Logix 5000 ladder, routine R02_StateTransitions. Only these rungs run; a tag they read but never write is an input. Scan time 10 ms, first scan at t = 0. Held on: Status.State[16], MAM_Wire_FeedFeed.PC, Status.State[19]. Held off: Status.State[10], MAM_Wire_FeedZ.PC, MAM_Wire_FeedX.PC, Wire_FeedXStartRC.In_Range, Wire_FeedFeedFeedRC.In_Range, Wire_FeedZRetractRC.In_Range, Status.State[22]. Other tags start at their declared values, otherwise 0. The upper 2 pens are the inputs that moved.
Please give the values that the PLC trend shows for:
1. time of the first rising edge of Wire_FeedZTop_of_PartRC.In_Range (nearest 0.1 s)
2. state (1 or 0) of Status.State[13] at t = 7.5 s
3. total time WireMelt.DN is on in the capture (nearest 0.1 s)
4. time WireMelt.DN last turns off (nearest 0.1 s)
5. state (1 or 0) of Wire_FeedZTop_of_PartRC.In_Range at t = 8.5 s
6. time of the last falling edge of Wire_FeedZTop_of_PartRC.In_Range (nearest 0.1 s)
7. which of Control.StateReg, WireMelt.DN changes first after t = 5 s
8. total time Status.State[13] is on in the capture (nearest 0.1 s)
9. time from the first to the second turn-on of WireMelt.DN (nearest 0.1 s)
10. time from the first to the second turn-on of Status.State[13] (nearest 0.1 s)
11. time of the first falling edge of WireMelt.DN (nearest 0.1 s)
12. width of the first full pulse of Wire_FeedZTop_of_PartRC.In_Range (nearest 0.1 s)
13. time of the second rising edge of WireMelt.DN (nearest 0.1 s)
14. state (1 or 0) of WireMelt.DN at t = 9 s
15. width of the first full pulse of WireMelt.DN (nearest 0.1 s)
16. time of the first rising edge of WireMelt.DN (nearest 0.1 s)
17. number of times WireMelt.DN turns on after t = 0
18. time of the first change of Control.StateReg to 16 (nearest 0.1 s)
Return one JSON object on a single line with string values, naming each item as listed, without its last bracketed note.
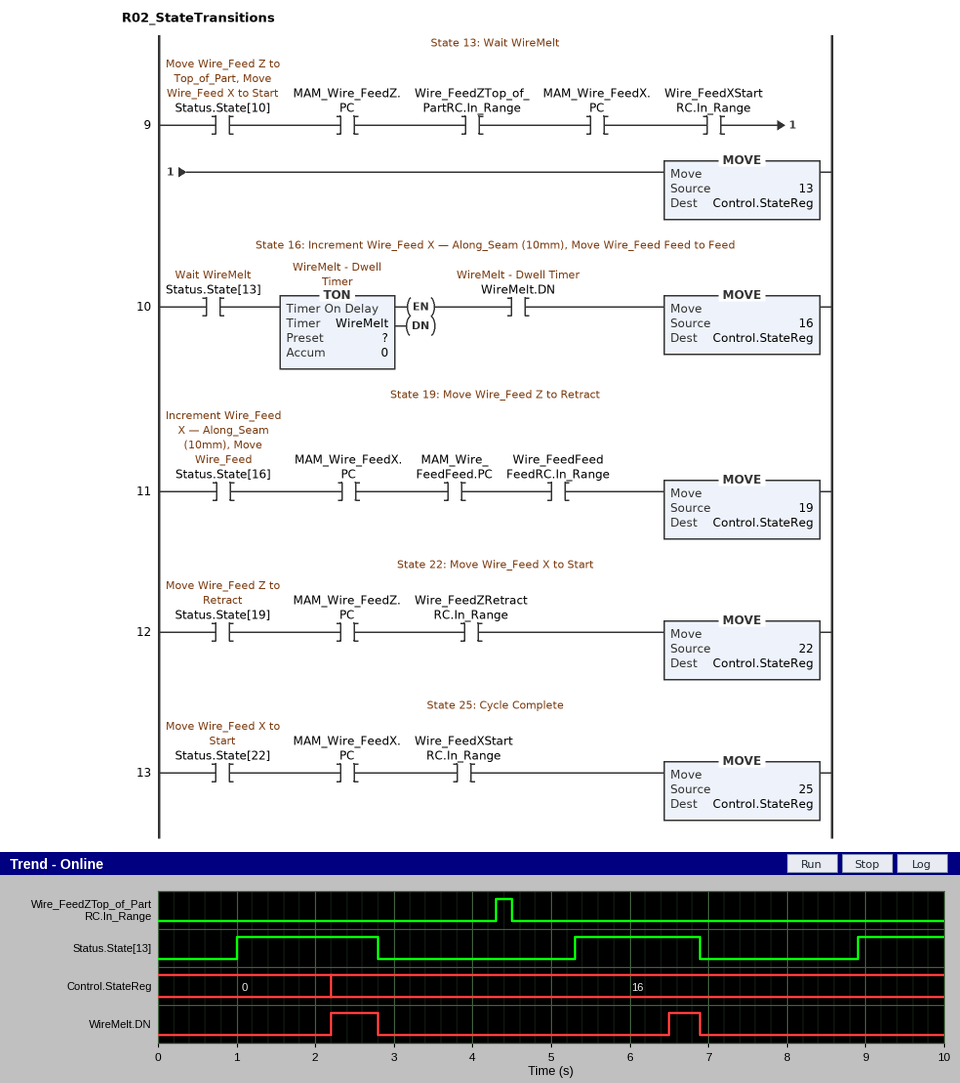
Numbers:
{"time of the first rising edge of Wire_FeedZTop_of_PartRC.In_Range": "4.3 s", "state (1 or 0) of Status.State[13] at t = 7.5 s": "0", "total time WireMelt.DN is on in the capture": "1.0 s", "time WireMelt.DN last turns off": "6.9 s", "state (1 or 0) of Wire_FeedZTop_of_PartRC.In_Range at t = 8.5 s": "0", "time of the last falling edge of Wire_FeedZTop_of_PartRC.In_Range": "4.5 s", "which of Control.StateReg, WireMelt.DN changes first after t = 5 s": "WireMelt.DN", "total time Status.State[13] is on in the capture": "4.5 s", "time from the first to the second turn-on of WireMelt.DN": "4.3 s", "time from the first to the second turn-on of Status.State[13]": "4.3 s", "time of the first falling edge of WireMelt.DN": "2.8 s", "width of the first full pulse of Wire_FeedZTop_of_PartRC.In_Range": "0.2 s", "time of the second rising edge of WireMelt.DN": "6.5 s", "state (1 or 0) of WireMelt.DN at t = 9 s": "0", "width of the first full pulse of WireMelt.DN": "0.6 s", "time of the first rising edge of WireMelt.DN": "2.2 s", "number of times WireMelt.DN turns on after t = 0": "2", "time of the first change of Control.StateReg to 16": "2.2 s"}
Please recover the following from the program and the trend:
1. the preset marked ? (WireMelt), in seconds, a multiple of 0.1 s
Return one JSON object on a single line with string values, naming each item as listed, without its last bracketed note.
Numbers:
{"the preset marked ? (WireMelt), in seconds, a multiple of 0.1 s": "1.2 s"}
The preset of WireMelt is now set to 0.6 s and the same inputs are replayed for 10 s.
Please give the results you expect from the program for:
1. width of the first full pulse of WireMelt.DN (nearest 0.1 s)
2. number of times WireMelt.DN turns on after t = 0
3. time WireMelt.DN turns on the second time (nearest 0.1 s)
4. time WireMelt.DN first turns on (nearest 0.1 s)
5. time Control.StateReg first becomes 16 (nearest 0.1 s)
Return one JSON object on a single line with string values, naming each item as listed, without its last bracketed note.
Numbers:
{"width of the first full pulse of WireMelt.DN": "1.2 s", "number of times WireMelt.DN turns on after t = 0": "3", "time WireMelt.DN turns on the second time": "5.9 s", "time WireMelt.DN first turns on": "1.6 s", "time Control.StateReg first becomes 16": "1.6 s"}
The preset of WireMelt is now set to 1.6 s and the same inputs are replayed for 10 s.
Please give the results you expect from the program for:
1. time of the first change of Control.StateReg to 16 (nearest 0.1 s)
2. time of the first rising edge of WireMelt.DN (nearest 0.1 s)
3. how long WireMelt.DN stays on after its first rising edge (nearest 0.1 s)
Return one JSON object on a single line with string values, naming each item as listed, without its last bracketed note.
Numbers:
{"time of the first change of Control.StateReg to 16": "2.6 s", "time of the first rising edge of WireMelt.DN": "2.6 s", "how long WireMelt.DN stays on after its first rising edge": "0.2 s"}
